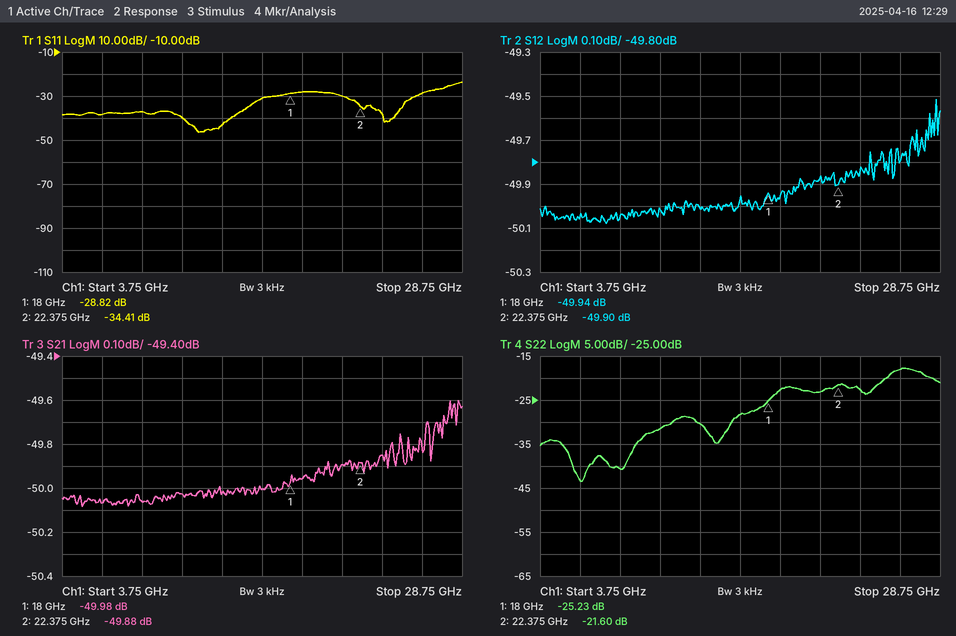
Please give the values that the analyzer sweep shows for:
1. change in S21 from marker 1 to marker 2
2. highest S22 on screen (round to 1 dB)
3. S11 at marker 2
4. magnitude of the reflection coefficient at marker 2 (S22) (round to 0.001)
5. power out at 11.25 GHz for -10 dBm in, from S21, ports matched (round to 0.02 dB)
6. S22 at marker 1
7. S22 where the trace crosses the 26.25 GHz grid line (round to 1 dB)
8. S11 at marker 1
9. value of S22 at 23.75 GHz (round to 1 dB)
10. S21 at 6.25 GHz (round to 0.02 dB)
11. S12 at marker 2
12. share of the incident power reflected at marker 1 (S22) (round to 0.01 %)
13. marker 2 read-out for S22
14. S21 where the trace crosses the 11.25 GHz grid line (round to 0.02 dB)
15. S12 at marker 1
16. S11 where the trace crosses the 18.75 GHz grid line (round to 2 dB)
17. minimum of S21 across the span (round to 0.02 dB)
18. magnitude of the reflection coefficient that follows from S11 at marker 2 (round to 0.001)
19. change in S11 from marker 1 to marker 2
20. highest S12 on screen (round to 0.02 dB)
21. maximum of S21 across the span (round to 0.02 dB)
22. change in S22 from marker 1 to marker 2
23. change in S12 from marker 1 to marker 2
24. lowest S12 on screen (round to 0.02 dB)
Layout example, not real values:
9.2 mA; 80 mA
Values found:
0.10 dB; -18 dB; -34.41 dB; 0.083; -60.02 dBm; -25.23 dB; -18 dB; -28.82 dB; -23 dB; -50.06 dB; -49.90 dB; 0.30 %; -21.60 dB; -50.02 dB; -49.94 dB; -28 dB; -50.08 dB; 0.019; -5.59 dB; -49.52 dB; -49.60 dB; 3.63 dB; 0.04 dB; -50.08 dB
